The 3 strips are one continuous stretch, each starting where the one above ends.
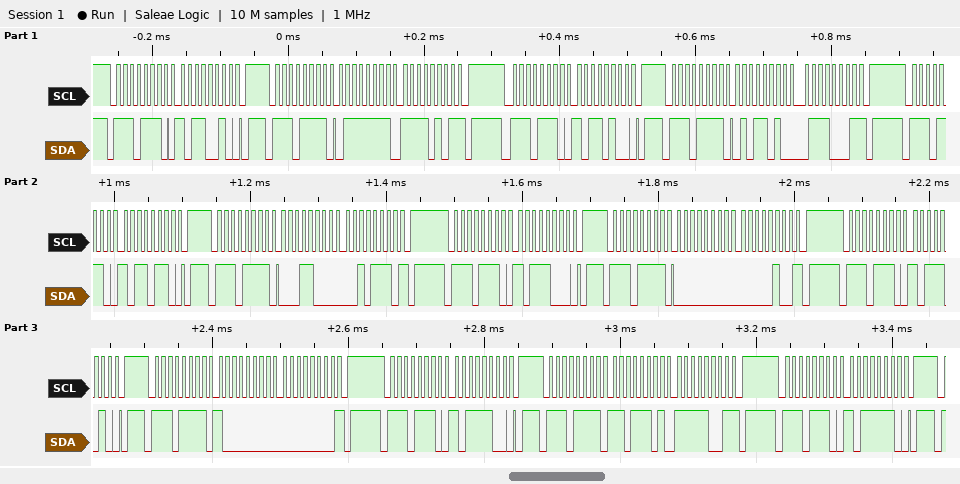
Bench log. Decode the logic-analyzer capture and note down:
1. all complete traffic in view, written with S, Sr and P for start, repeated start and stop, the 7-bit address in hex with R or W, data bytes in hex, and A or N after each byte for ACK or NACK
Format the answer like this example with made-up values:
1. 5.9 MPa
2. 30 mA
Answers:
1. S 77W A B2 A P S 77R A 7F A F5 N P S 77W A B4 A P S 77R A 5A A 71 N P S 77W A B6 A P S 77R A 18 A 2E N P S 77W A B8 A P S 77R A 00 A 04 N P S 77W A BA A P S 77R A 80 A 00 N P S 77W A BC A P S 77R A DD A F9 N P S 77W A BE A P
